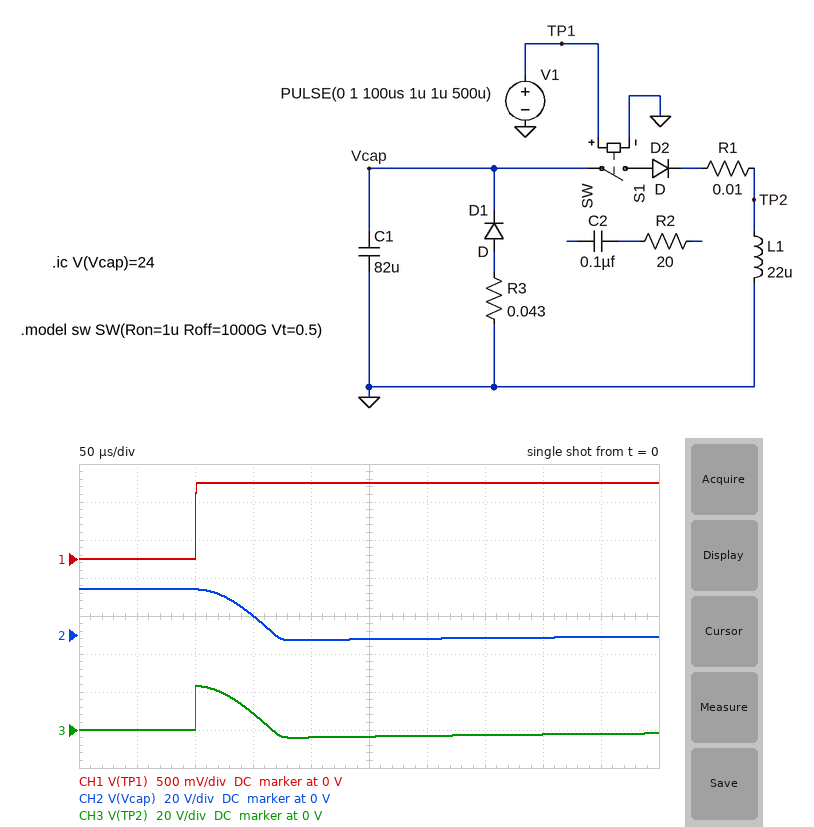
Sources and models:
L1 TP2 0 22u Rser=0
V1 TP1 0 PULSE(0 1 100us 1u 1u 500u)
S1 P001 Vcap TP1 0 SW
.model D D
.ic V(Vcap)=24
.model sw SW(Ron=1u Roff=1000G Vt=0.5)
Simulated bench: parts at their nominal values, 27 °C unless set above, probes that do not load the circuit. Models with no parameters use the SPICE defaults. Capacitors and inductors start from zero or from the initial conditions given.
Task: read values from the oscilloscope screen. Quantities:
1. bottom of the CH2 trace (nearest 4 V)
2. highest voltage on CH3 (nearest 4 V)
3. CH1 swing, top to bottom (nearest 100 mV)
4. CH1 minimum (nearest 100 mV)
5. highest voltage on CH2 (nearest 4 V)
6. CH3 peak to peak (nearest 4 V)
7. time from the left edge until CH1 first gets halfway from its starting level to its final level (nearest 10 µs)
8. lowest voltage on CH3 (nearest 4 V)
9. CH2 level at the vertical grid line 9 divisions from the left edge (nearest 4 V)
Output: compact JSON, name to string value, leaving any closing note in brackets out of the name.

{"bottom of the CH2 trace": "-4 V", "highest voltage on CH3": "24 V", "CH1 swing, top to bottom": "1.0 V", "CH1 minimum": "0 V", "highest voltage on CH2": "24 V", "CH3 peak to peak": "28 V", "time from the left edge until CH1 first gets halfway from its starting level to its final level": "100 µs", "lowest voltage on CH3": "-4 V", "CH2 level at the vertical grid line 9 divisions from the left edge": "0 V"}
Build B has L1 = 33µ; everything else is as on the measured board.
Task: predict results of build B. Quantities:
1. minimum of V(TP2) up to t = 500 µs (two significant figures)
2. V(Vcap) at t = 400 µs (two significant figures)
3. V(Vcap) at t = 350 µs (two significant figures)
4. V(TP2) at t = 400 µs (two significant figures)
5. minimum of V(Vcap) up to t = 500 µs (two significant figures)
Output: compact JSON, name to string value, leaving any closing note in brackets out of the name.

{"minimum of V(TP2) up to t = 500 µs": "-3.7 V", "V(Vcap) at t = 400 µs": "-1.6 V", "V(Vcap) at t = 350 µs": "-1.8 V", "V(TP2) at t = 400 µs": "-2.6 V", "minimum of V(Vcap) up to t = 500 µs": "-2.4 V"}
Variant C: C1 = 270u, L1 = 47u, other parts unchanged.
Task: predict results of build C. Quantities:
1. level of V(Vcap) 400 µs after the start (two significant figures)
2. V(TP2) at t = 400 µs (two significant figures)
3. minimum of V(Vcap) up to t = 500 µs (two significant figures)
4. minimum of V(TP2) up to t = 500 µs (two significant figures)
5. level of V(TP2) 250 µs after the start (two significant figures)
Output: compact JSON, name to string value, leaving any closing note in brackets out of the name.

{"level of V(Vcap) 400 µs after the start": "-2.9 V", "V(TP2) at t = 400 µs": "-4.2 V", "minimum of V(Vcap) up to t = 500 µs": "-3.1 V", "minimum of V(TP2) up to t = 500 µs": "-4.5 V", "level of V(TP2) 250 µs after the start": "5.2 V"}
